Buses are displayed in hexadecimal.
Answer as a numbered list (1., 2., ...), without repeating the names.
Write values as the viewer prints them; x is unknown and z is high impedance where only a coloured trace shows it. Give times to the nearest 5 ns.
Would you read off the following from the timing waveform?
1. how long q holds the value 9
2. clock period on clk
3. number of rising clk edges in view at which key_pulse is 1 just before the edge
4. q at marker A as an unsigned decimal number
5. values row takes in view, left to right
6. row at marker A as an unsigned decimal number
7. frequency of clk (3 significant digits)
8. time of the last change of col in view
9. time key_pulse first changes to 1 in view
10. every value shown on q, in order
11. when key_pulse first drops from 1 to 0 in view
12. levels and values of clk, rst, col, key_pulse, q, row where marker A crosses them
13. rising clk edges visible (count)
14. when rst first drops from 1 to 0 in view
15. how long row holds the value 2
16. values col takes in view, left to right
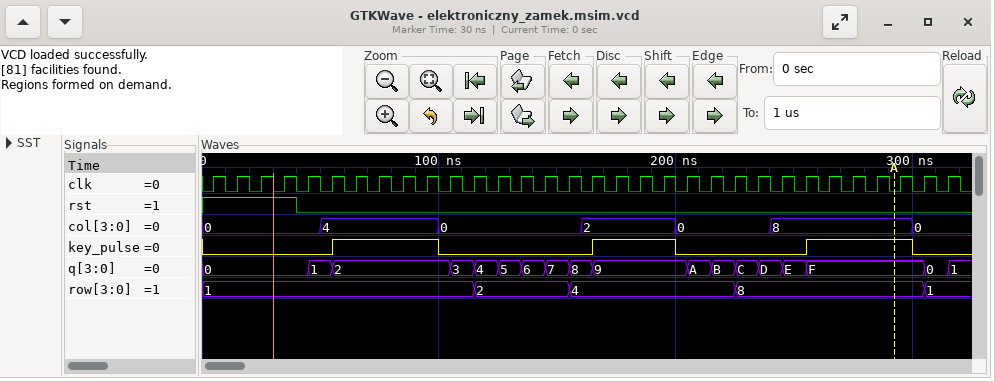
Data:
1. 40 ns
2. 10 ns
3. 11
4. 15
5. 1, 2, 4, 8, 1
6. 8
7. 100 MHz
8. 300 ns
9. 55 ns
10. 0, 1, 2, 3, 4, 5, 6, 7, 8, 9, A, B, C, D, E, F, 0, 1
11. 100 ns
12. clk=0, rst=0, col=8, key_pulse=1, q=F, row=8
13. 32
14. 40 ns
15. 40 ns
16. 0, 4, 0, 2, 0, 8, 0
